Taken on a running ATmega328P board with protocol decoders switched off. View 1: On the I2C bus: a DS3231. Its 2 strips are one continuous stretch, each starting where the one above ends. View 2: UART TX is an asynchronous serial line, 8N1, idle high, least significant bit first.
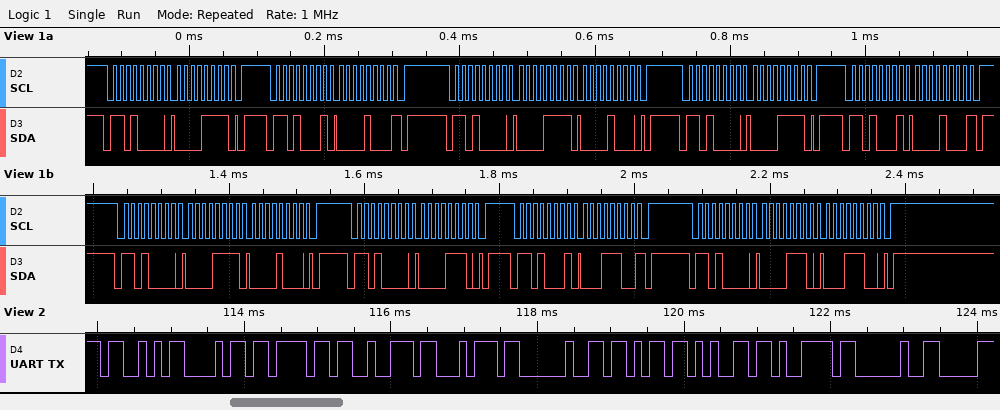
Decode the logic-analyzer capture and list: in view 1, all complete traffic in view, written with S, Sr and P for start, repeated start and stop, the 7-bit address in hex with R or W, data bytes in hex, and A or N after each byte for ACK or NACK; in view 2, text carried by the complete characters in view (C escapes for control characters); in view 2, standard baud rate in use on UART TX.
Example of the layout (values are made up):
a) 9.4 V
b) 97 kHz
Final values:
a) S 68W A 0F A P S 68R A 08 N P S 68W A 0F A 08 A P S 68W A 0F A P S 68R A 08 N P S 68W A 0F A 08 A P S 68W A 0E A P S 68R A 1C N P S 68W A 0E A 1C A P
b) "Short key "
c) 9600 baud
